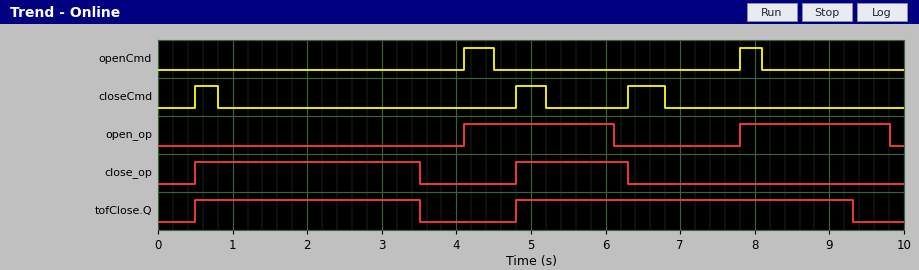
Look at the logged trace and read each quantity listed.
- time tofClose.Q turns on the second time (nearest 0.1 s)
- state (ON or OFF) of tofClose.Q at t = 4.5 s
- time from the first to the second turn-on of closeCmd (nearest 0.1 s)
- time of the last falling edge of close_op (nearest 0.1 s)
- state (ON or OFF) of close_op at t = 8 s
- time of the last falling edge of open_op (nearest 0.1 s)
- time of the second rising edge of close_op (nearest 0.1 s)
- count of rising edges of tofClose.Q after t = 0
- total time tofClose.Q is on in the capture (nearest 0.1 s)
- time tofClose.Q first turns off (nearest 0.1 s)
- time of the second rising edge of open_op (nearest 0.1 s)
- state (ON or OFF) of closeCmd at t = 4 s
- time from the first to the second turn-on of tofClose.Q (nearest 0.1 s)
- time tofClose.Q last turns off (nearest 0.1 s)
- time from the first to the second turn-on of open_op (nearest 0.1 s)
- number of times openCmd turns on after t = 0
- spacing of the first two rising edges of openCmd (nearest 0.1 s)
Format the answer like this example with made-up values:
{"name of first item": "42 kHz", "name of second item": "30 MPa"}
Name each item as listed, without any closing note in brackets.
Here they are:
{"time tofClose.Q turns on the second time": "4.8 s", "state (ON or OFF) of tofClose.Q at t = 4.5 s": "OFF", "time from the first to the second turn-on of closeCmd": "4.3 s", "time of the last falling edge of close_op": "6.3 s", "state (ON or OFF) of close_op at t = 8 s": "OFF", "time of the last falling edge of open_op": "9.8 s", "time of the second rising edge of close_op": "4.8 s", "count of rising edges of tofClose.Q after t = 0": "2", "total time tofClose.Q is on in the capture": "7.5 s", "time tofClose.Q first turns off": "3.5 s", "time of the second rising edge of open_op": "7.8 s", "state (ON or OFF) of closeCmd at t = 4 s": "OFF", "time from the first to the second turn-on of tofClose.Q": "4.3 s", "time tofClose.Q last turns off": "9.3 s", "time from the first to the second turn-on of open_op": "3.7 s", "number of times openCmd turns on after t = 0": "2", "spacing of the first two rising edges of openCmd": "3.7 s"}
